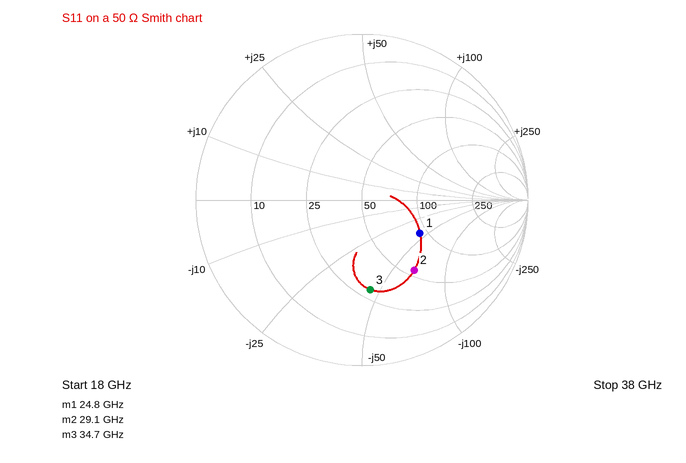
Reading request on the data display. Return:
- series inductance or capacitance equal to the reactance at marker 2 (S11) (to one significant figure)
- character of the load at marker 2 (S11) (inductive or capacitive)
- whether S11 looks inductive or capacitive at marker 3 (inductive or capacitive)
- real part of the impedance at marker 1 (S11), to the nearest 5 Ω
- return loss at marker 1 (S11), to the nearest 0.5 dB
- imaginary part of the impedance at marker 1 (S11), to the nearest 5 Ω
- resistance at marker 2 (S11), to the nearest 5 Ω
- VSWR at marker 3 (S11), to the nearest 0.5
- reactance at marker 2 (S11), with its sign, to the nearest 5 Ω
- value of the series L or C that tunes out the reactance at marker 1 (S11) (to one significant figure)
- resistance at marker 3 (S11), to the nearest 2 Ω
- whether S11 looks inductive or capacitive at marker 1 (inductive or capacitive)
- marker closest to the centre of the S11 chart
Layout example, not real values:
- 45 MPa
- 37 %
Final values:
- 80 fF
- capacitive
- capacitive
- 90 Ω
- 8.0 dB
- -45 Ω
- 55 Ω
- 3.5
- -65 Ω
- 300 pH
- 30 Ω
- capacitive
- marker 1
